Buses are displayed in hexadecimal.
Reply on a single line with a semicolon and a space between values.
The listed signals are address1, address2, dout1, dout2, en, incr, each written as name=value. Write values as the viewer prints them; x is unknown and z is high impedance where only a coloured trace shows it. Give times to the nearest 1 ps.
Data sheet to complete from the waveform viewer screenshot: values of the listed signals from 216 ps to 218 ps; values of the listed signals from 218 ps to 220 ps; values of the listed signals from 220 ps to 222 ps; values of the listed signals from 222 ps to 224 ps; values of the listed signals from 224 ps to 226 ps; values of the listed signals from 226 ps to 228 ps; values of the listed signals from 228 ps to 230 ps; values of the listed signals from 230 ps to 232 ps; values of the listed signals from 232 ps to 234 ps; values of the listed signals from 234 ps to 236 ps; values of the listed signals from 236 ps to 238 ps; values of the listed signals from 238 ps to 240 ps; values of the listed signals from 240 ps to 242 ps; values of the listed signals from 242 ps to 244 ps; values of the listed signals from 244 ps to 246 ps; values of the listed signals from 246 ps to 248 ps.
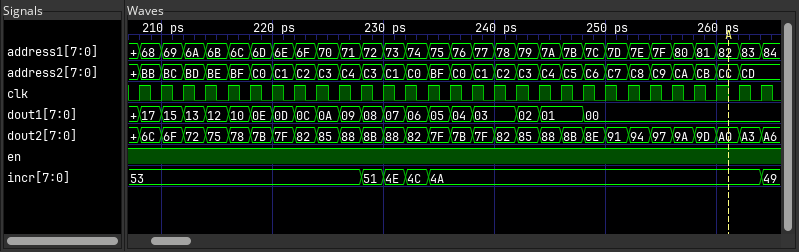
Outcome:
address1=6C, address2=BF, dout1=10, dout2=78, en=1, incr=53; address1=6D, address2=C0, dout1=0E, dout2=7B, en=1, incr=53; address1=6E, address2=C1, dout1=0D, dout2=7F, en=1, incr=53; address1=6F, address2=C2, dout1=0C, dout2=82, en=1, incr=53; address1=70, address2=C3, dout1=0A, dout2=85, en=1, incr=53; address1=71, address2=C4, dout1=09, dout2=88, en=1, incr=53; address1=72, address2=C3, dout1=08, dout2=8B, en=1, incr=51; address1=73, address2=C1, dout1=07, dout2=88, en=1, incr=4E; address1=74, address2=C0, dout1=06, dout2=82, en=1, incr=4C; address1=75, address2=BF, dout1=05, dout2=7F, en=1, incr=4A; address1=76, address2=C0, dout1=04, dout2=7B, en=1, incr=4A; address1=77, address2=C1, dout1=03, dout2=7F, en=1, incr=4A; address1=78, address2=C2, dout1=03, dout2=82, en=1, incr=4A; address1=79, address2=C3, dout1=02, dout2=85, en=1, incr=4A; address1=7A, address2=C4, dout1=01, dout2=88, en=1, incr=4A; address1=7B, address2=C5, dout1=01, dout2=8B, en=1, incr=4A
